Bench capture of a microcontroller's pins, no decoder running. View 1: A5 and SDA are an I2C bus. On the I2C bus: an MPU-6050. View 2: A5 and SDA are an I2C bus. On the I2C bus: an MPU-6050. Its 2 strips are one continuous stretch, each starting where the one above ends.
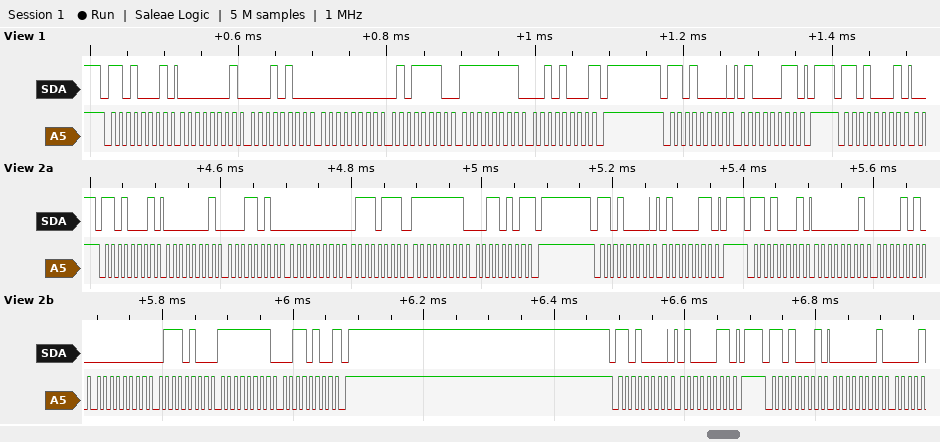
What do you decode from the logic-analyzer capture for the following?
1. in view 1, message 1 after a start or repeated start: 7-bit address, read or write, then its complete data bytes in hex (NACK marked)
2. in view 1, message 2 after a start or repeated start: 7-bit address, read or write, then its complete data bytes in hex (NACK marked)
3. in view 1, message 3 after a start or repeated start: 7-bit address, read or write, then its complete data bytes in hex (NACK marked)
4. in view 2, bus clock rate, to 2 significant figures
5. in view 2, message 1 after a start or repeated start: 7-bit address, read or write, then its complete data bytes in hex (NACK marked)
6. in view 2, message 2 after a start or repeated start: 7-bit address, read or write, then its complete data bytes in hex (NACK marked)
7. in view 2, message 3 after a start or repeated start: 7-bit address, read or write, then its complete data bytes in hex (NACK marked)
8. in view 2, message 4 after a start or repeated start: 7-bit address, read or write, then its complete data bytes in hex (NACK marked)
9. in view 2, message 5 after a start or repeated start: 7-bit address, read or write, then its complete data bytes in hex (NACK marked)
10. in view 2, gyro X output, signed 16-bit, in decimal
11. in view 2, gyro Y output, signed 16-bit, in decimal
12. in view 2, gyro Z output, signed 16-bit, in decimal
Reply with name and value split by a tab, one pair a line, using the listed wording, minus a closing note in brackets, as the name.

in view 1, message 1 after a start or repeated start: 7-bit address, read or write, then its complete data bytes in hex	0x68 read: 01 14 00 5E FF 28 NACK
in view 1, message 2 after a start or repeated start: 7-bit address, read or write, then its complete data bytes in hex	0x68 write: 43
in view 1, message 3 after a start or repeated start: 7-bit address, read or write, then its complete data bytes in hex	0x68 read
in view 2, bus clock rate, to 2 significant figures	100 kHz
in view 2, message 1 after a start or repeated start: 7-bit address, read or write, then its complete data bytes in hex	0x68 read: 01 1A 00 77 FF 35 NACK
in view 2, message 2 after a start or repeated start: 7-bit address, read or write, then its complete data bytes in hex	0x68 write: 43
in view 2, message 3 after a start or repeated start: 7-bit address, read or write, then its complete data bytes in hex	0x68 read: 01 0A 00 74 FF 34 NACK
in view 2, message 4 after a start or repeated start: 7-bit address, read or write, then its complete data bytes in hex	0x68 write: 43
in view 2, message 5 after a start or repeated start: 7-bit address, read or write, then its complete data bytes in hex	0x68 read: 01
in view 2, gyro X output, signed 16-bit, in decimal	266
in view 2, gyro Y output, signed 16-bit, in decimal	116
in view 2, gyro Z output, signed 16-bit, in decimal	-204
